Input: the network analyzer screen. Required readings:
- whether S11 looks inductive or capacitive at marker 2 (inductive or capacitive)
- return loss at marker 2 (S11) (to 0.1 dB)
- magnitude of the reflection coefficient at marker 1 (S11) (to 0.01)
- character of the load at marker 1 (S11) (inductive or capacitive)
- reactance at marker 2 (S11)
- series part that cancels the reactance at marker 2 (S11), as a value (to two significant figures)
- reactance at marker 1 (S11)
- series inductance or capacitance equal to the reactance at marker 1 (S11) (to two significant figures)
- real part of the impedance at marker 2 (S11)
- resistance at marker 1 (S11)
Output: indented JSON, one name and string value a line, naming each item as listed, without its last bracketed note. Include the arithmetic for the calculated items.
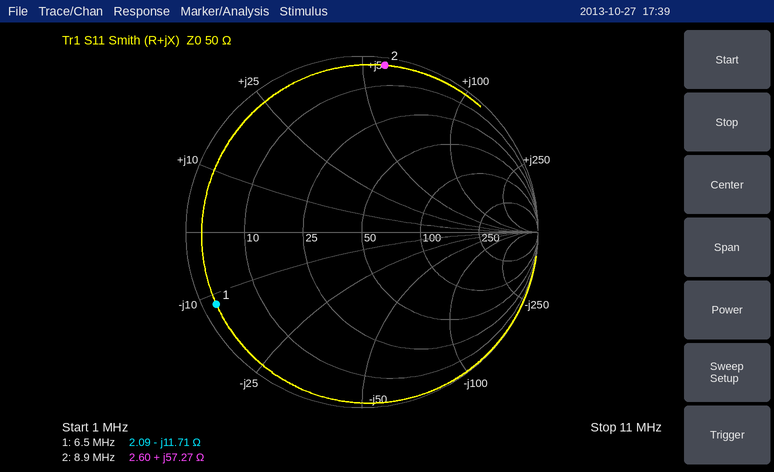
{
  "whether S11 looks inductive or capacitive at marker 2": "inductive",
  "return loss at marker 2 (S11)": "0.4 dB",
  "magnitude of the reflection coefficient at marker 1 (S11)": "0.92",
  "character of the load at marker 1 (S11)": "capacitive",
  "reactance at marker 2": "+57.27 Ω",
  "series part that cancels the reactance at marker 2 (S11), as a value": "C = 1/(2π × 8.9 MHz × 57.27 Ω) ≈ 312 pF, so 310 pF to two significant figures",
  "reactance at marker 1": "-11.71 Ω",
  "series inductance or capacitance equal to the reactance at marker 1 (S11)": "C = 1/(2π × 6.5 MHz × 11.71 Ω) ≈ 2.1 nF",
  "real part of the impedance at marker 2": "2.60 Ω",
  "resistance at marker 1": "2.09 Ω"
}
